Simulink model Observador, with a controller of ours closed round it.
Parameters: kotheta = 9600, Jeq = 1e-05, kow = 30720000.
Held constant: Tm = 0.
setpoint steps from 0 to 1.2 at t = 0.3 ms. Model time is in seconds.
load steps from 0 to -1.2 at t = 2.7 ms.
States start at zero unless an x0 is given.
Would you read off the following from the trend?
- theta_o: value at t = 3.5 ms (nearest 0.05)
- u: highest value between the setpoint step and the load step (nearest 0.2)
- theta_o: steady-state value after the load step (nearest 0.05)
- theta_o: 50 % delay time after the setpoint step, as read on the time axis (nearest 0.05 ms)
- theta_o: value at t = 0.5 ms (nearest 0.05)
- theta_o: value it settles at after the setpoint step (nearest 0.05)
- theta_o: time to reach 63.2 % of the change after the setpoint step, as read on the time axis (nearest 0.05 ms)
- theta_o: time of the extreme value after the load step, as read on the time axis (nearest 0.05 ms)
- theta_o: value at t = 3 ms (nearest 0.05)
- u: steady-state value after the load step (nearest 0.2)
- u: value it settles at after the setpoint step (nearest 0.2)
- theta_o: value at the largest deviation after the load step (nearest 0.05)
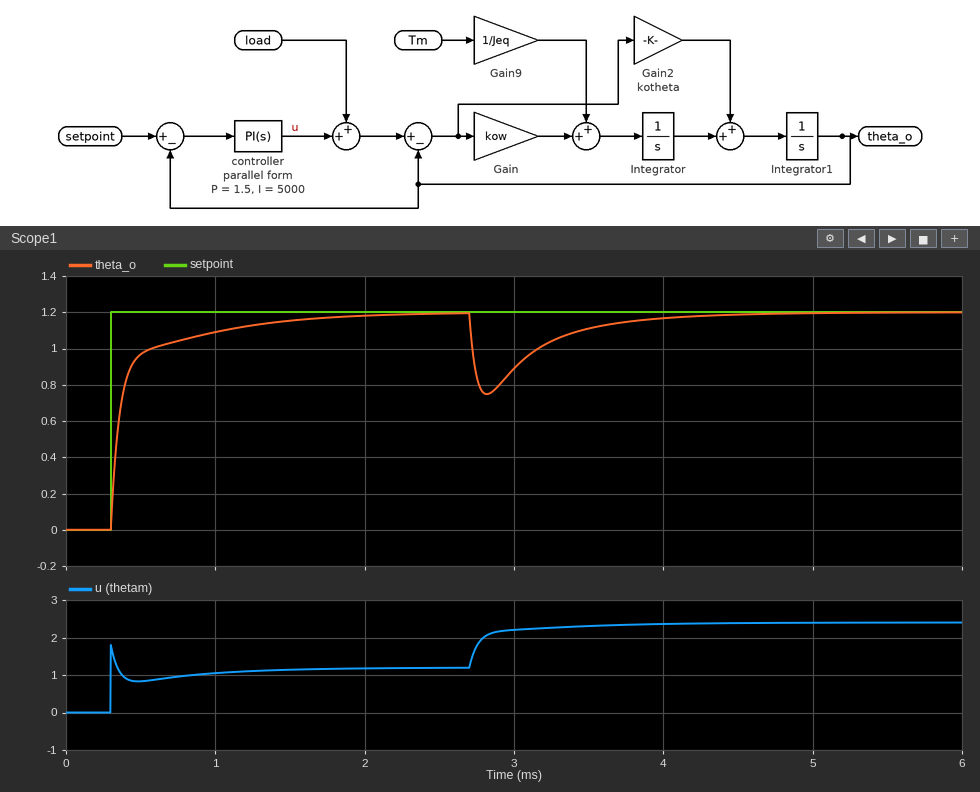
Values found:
1.10
1.8
1.20
0.35 ms
0.95
1.20
0.40 ms
2.80 ms
0.90
2.4
1.2
0.75
